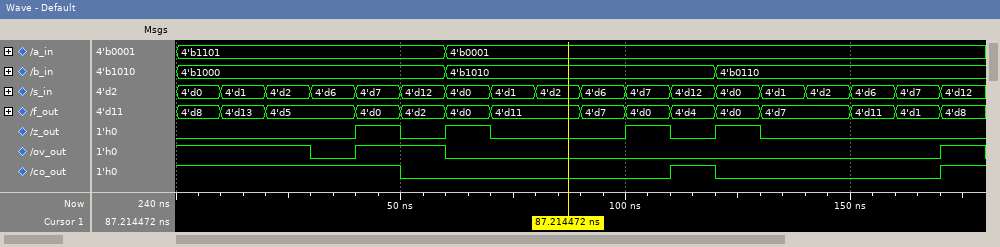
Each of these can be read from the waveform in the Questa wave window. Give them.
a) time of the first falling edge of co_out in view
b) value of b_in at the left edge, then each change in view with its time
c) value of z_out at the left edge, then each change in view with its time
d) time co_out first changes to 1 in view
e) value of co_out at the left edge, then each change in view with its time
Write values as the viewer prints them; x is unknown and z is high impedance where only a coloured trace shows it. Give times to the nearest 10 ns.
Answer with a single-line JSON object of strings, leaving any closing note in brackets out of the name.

{"time of the first falling edge of co_out in view": "50 ns", "value of b_in at the left edge, then each change in view with its time": "4'b1000, 4'b1010 at 60 ns, 4'b0110 at 120 ns", "value of z_out at the left edge, then each change in view with its time": "0, 1 at 40 ns, 0 at 50 ns, 1 at 60 ns, 0 at 70 ns, 1 at 100 ns, 0 at 110 ns, 1 at 120 ns, 0 at 130 ns", "time co_out first changes to 1 in view": "110 ns", "value of co_out at the left edge, then each change in view with its time": "1, 0 at 50 ns, 1 at 110 ns, 0 at 120 ns, 1 at 170 ns"}
